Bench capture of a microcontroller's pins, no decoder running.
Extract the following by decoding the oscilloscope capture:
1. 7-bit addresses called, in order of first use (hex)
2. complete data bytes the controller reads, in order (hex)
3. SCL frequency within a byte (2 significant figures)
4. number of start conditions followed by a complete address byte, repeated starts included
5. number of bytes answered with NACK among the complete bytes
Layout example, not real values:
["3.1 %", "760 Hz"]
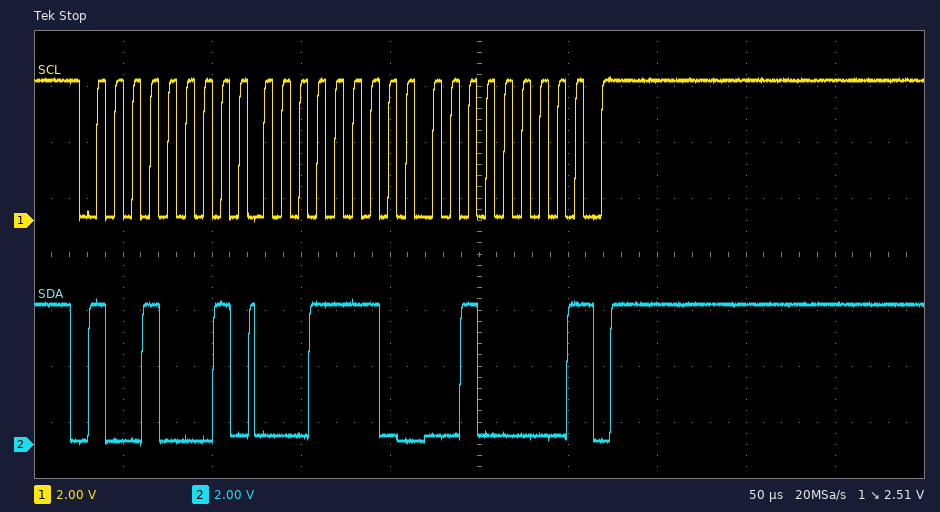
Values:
["0x48", "1E 20", "100 kHz", "1", "1"]
